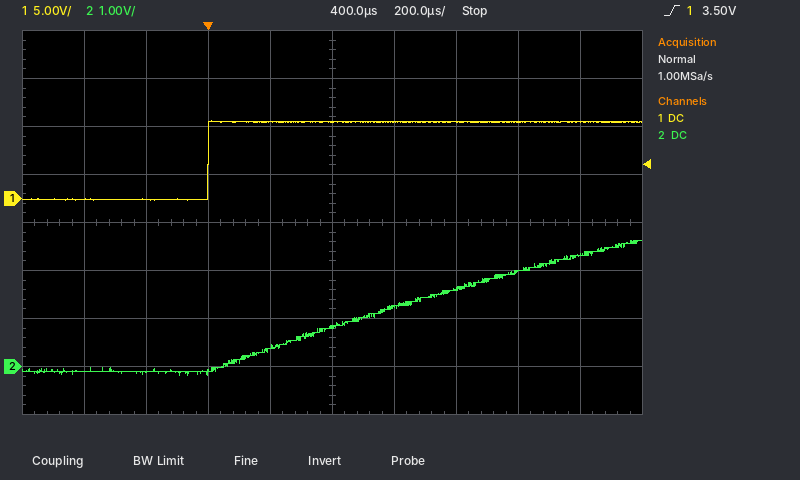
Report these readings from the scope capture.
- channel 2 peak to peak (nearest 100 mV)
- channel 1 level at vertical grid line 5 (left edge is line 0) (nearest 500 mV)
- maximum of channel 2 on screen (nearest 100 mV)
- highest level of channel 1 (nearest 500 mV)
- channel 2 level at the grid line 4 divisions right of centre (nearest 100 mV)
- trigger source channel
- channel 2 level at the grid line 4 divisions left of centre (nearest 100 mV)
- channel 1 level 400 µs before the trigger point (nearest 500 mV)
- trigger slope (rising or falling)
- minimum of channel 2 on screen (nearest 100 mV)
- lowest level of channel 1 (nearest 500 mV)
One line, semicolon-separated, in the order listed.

2.8 V; 8.0 V; 2.6 V; 8.0 V; 2.3 V; channel 1; -100 mV; 0.0 V; rising; -200 mV; 0.0 V
